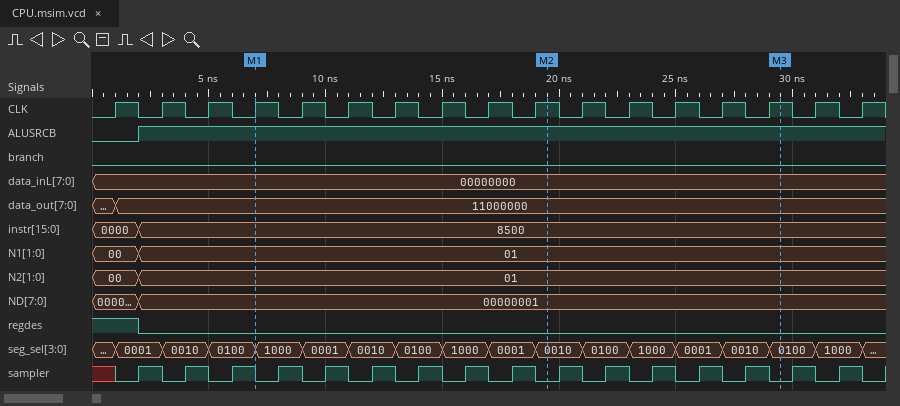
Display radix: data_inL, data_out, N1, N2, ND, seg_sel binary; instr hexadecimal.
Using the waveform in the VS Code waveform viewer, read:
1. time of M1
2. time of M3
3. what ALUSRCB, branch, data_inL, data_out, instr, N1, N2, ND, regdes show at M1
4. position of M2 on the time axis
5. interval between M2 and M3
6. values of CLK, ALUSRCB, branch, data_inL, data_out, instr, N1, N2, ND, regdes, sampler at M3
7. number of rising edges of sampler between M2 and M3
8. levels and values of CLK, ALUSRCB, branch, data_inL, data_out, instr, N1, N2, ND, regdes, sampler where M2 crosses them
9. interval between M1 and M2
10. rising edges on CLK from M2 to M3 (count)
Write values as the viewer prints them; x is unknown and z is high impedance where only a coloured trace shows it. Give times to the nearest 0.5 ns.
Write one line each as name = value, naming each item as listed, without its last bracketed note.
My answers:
time of M1 = 7 ns
time of M3 = 29.5 ns
what ALUSRCB, branch, data_inL, data_out, instr, N1, N2, ND, regdes show at M1 = ALUSRCB=1, branch=0, data_inL=00000000, data_out=11000000, instr=8500, N1=01, N2=01, ND=00000001, regdes=0
position of M2 on the time axis = 19.5 ns
interval between M2 and M3 = 10 ns
values of CLK, ALUSRCB, branch, data_inL, data_out, instr, N1, N2, ND, regdes, sampler at M3 = CLK=1, ALUSRCB=1, branch=0, data_inL=00000000, data_out=11000000, instr=8500, N1=01, N2=01, ND=00000001, regdes=0, sampler=0
number of rising edges of sampler between M2 and M3 = 5
levels and values of CLK, ALUSRCB, branch, data_inL, data_out, instr, N1, N2, ND, regdes, sampler where M2 crosses them = CLK=1, ALUSRCB=1, branch=0, data_inL=00000000, data_out=11000000, instr=8500, N1=01, N2=01, ND=00000001, regdes=0, sampler=0
interval between M1 and M2 = 12.5 ns
rising edges on CLK from M2 to M3 = 5
